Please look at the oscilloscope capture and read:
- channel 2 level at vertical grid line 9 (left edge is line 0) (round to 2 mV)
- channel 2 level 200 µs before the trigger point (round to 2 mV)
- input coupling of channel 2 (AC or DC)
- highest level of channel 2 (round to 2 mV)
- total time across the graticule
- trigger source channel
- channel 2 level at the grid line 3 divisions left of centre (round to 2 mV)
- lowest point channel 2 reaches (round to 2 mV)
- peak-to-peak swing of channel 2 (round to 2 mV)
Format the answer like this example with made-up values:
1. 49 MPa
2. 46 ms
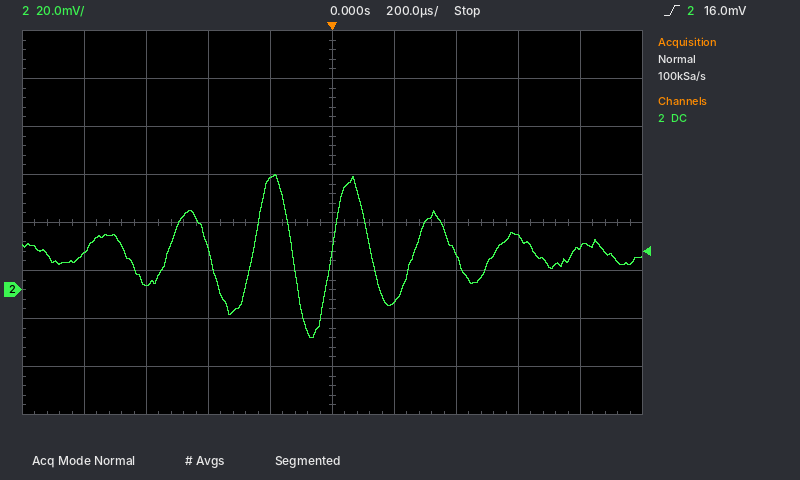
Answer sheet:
1. 18 mV
2. 46 mV
3. DC
4. 48 mV
5. 2 ms
6. channel 2
7. 2 mV
8. -20 mV
9. 68 mV
